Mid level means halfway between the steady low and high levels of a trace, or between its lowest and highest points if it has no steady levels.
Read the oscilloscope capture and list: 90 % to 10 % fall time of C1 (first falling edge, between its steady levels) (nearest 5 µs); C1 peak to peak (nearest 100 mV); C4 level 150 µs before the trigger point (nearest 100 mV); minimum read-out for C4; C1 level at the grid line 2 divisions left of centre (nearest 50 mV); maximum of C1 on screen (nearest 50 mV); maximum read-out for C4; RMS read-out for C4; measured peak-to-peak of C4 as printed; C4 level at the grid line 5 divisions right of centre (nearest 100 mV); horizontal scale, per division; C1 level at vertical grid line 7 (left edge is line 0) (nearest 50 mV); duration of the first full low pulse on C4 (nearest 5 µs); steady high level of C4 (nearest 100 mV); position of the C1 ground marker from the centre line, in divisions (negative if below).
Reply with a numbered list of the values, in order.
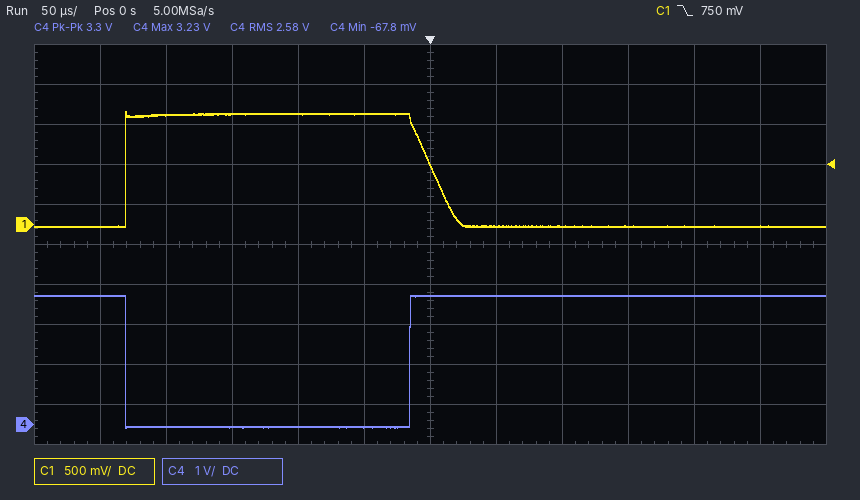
1. 30 µs
2. 1.40 V
3. -100 mV
4. -67.8 mV
5. 1.40 V
6. 1.40 V
7. 3.23 V
8. 2.58 V
9. 3.3 V
10. 3.2 V
11. 50 µs
12. 0 mV
13. 215 µs
14. 3.2 V
15. +0.5 div
